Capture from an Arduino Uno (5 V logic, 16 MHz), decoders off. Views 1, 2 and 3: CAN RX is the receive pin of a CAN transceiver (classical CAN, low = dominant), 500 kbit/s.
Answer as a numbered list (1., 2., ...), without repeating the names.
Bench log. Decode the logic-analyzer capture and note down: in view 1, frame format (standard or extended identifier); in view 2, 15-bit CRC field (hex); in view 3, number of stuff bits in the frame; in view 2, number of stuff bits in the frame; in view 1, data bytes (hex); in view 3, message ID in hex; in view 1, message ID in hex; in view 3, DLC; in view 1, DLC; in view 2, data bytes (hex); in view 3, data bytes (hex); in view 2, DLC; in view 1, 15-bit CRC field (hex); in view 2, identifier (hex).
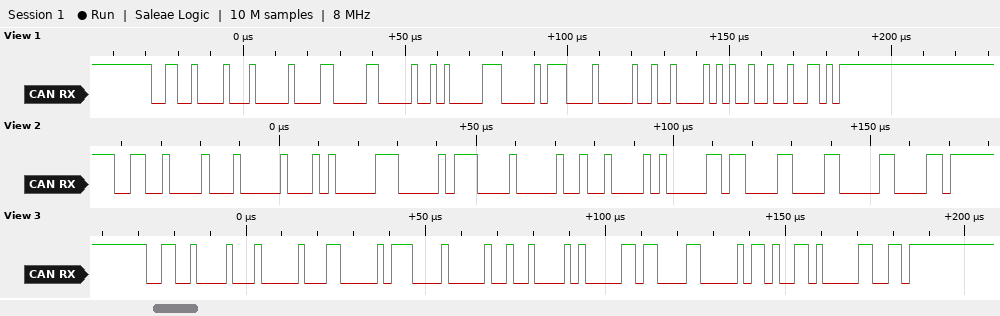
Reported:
1. standard
2. 0x1821
3. 6
4. 6
5. 03 04 05 06 07 08 09 0A
6. 0x321
7. 0x321
8. 8
9. 8
10. 05 06 07 08 09 0A 0B 0C
11. 06 07 08 09 0A 0B 0C 0D
12. 8
13. 0x4926
14. 0x321
